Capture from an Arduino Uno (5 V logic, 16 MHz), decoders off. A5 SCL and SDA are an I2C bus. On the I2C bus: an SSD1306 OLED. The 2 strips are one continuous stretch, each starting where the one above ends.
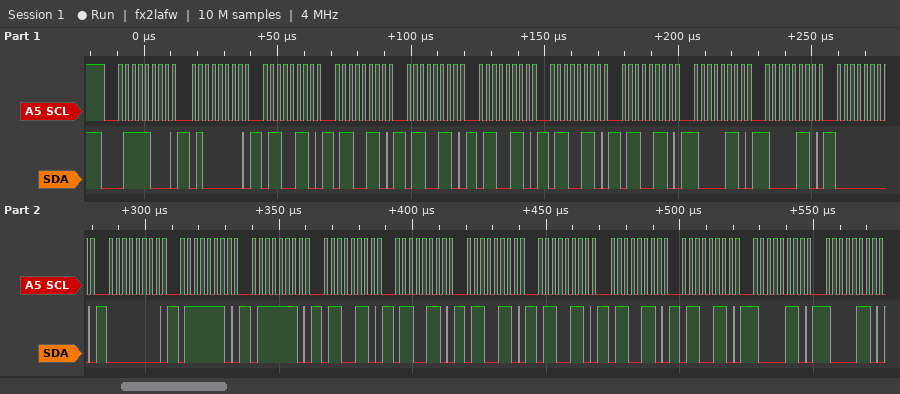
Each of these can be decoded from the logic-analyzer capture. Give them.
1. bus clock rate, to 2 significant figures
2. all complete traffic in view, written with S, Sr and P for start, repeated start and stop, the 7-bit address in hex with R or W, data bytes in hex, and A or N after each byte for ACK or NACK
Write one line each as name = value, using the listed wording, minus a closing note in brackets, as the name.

bus clock rate, to 2 significant figures = 400 kHz
all complete traffic in view, written with S, Sr and P for start, repeated start and stop, the 7-bit address in hex with R or W, data bytes in hex, and A or N after each byte for ACK or NACK = S 3CW A 40 A 66 A 66 A 66 A 66 A 66 A 66 A 86 A 86 A 00 A 00 A 7E A 7E A 66 A 66 A 66 A 66 A 66 A 66 A 86 A 86 A
